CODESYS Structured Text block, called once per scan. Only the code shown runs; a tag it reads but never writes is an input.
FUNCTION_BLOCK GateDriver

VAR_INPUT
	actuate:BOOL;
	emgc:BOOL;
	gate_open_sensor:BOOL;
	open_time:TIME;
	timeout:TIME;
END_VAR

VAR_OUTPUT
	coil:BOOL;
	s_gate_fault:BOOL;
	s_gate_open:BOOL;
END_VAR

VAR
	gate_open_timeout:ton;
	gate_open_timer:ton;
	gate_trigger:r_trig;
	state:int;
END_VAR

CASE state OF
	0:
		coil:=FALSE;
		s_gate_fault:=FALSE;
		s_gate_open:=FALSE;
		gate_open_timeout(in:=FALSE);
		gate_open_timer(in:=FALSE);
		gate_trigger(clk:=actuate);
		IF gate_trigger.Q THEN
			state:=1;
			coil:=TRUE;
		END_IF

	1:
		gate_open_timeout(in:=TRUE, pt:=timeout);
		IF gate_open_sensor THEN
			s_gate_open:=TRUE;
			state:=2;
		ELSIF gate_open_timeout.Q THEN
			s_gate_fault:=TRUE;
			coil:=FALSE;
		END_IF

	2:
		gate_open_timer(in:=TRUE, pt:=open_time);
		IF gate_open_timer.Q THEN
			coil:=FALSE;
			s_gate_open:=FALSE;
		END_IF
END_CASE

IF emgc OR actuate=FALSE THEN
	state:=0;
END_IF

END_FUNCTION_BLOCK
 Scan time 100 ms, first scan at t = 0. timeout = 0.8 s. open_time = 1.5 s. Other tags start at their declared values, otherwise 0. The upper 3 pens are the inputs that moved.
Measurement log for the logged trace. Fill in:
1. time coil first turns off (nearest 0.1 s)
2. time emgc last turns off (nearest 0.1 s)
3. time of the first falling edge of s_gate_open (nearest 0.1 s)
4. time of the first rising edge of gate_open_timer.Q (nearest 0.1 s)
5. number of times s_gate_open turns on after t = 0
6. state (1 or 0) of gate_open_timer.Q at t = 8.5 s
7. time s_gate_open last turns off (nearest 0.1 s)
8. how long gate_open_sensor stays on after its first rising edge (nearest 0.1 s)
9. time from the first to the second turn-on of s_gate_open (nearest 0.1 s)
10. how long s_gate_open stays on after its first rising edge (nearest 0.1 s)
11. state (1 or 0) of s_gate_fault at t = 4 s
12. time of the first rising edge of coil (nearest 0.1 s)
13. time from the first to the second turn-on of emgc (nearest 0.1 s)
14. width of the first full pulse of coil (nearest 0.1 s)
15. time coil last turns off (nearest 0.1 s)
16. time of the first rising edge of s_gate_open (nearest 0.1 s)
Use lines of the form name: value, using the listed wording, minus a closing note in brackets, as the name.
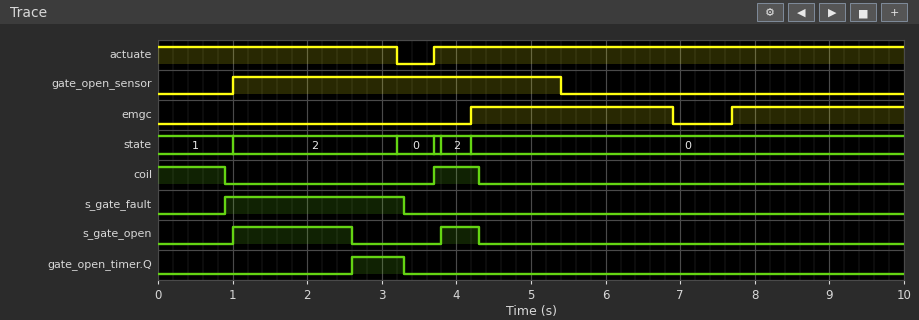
time coil first turns off: 0.9 s
time emgc last turns off: 6.9 s
time of the first falling edge of s_gate_open: 2.6 s
time of the first rising edge of gate_open_timer.Q: 2.6 s
number of times s_gate_open turns on after t = 0: 2
state (1 or 0) of gate_open_timer.Q at t = 8.5 s: 0
time s_gate_open last turns off: 4.3 s
how long gate_open_sensor stays on after its first rising edge: 4.4 s
time from the first to the second turn-on of s_gate_open: 2.8 s
how long s_gate_open stays on after its first rising edge: 1.6 s
state (1 or 0) of s_gate_fault at t = 4 s: 0
time of the first rising edge of coil: 3.7 s
time from the first to the second turn-on of emgc: 3.5 s
width of the first full pulse of coil: 0.6 s
time coil last turns off: 4.3 s
time of the first rising edge of s_gate_open: 1.0 s
